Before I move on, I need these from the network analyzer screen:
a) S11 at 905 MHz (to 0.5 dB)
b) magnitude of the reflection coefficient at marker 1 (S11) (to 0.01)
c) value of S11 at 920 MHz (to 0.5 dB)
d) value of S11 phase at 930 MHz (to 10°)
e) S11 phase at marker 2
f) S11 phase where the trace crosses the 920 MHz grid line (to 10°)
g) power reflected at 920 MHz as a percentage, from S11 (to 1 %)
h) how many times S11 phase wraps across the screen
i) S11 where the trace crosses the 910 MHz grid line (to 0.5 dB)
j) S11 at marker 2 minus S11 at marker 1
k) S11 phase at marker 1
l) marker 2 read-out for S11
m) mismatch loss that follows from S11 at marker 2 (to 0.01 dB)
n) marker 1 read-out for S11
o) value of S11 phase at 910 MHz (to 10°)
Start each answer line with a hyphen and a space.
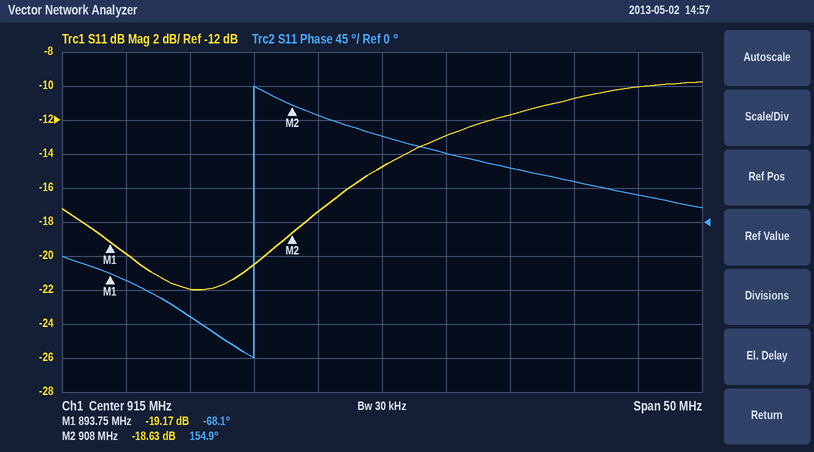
- -20.5 dB
- 0.11
- -13.0 dB
- 50°
- 154.9°
- 90°
- 5 %
- 1
- -17.5 dB
- 0.54 dB
- -68.1°
- -18.63 dB
- 0.06 dB
- -19.17 dB
- 140°
